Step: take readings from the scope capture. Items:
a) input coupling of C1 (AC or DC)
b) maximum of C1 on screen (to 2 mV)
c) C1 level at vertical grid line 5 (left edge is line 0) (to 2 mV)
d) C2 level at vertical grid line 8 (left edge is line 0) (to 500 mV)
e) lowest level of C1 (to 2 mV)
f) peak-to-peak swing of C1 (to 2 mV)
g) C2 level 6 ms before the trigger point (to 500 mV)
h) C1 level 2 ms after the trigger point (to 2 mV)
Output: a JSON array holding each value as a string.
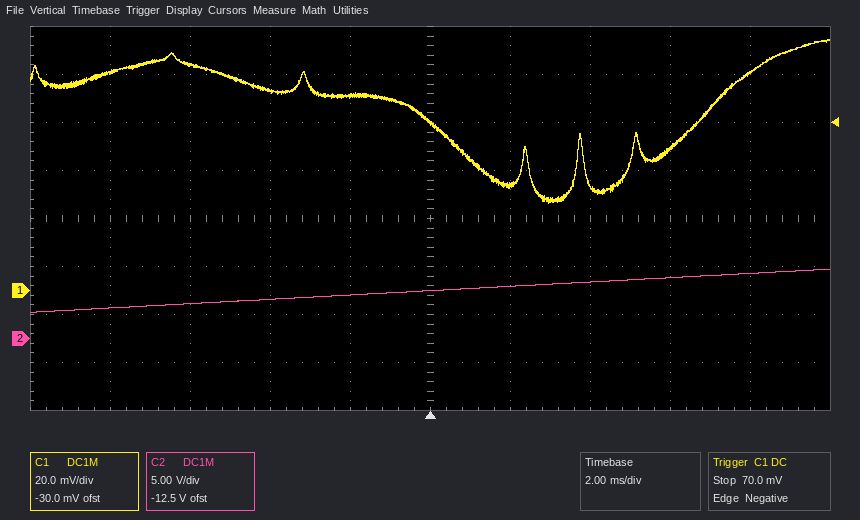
["DC", "104 mV", "70 mV", "6.5 V", "36 mV", "68 mV", "3.5 V", "44 mV"]
